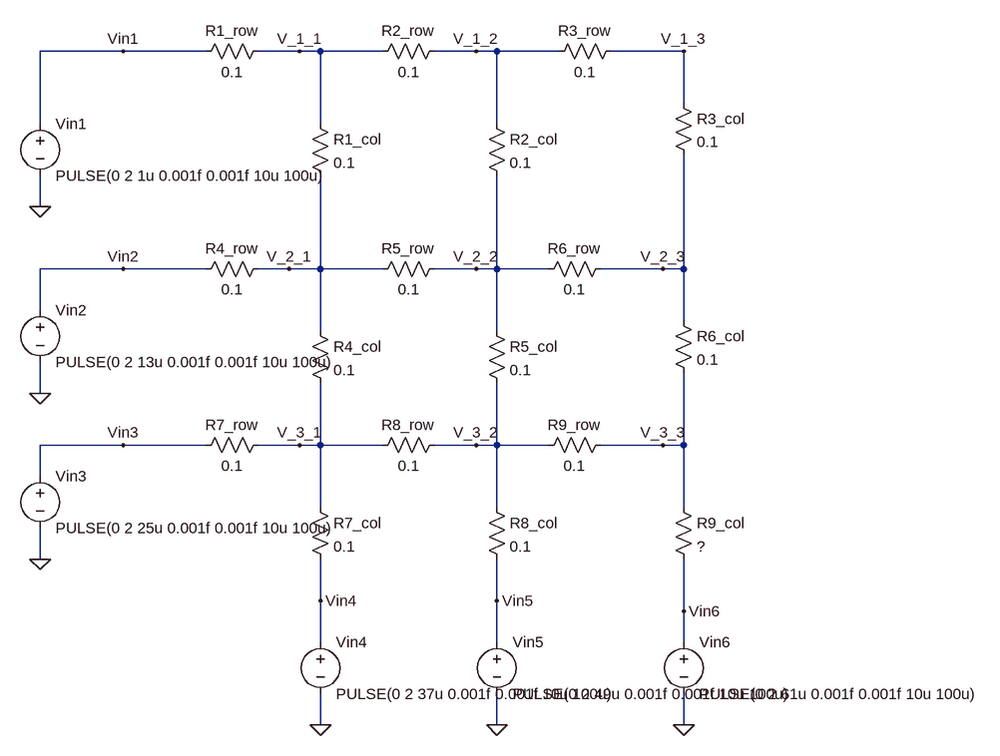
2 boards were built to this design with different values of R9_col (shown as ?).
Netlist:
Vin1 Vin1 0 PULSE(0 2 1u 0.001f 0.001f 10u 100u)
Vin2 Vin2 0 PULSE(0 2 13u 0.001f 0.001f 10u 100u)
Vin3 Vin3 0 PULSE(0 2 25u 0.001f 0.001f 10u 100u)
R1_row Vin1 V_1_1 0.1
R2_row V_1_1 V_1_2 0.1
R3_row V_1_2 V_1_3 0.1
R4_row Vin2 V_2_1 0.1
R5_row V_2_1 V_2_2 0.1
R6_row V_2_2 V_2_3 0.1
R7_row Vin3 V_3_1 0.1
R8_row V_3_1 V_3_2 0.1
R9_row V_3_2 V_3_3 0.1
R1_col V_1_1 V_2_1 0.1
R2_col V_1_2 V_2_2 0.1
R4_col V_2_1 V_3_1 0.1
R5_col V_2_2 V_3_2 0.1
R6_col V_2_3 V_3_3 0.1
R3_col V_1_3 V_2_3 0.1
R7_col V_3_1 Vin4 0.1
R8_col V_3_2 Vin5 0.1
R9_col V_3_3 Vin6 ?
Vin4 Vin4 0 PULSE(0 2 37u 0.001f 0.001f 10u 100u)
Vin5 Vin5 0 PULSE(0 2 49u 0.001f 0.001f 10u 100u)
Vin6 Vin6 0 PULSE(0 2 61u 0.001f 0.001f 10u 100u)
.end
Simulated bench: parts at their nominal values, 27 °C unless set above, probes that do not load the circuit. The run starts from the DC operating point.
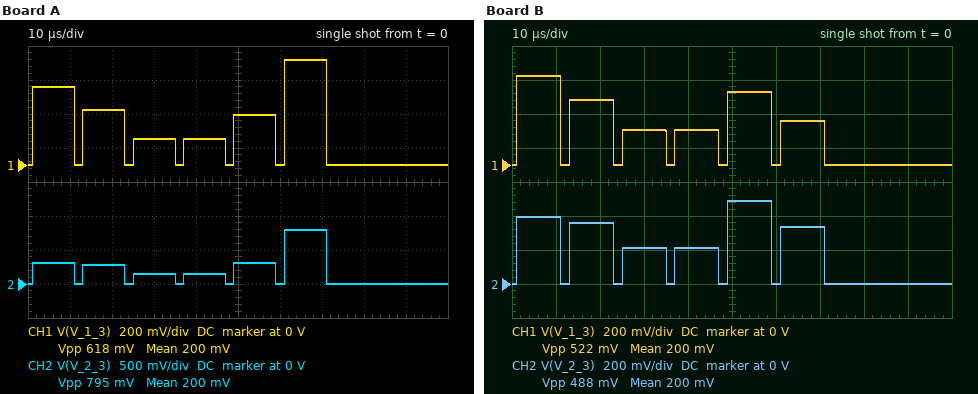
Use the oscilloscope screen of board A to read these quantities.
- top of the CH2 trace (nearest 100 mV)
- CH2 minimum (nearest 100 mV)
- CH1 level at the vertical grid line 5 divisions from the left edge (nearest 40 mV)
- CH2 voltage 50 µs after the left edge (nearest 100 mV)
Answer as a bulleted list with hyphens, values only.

- 800 mV
- 0 V
- 280 mV
- 300 mV
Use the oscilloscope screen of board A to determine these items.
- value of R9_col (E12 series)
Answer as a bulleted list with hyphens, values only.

- 0.056 Ω
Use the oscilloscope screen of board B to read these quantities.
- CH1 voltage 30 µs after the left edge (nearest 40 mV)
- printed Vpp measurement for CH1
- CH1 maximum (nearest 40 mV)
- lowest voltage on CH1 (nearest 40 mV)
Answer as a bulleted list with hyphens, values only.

- 200 mV
- 522 mV
- 520 mV
- 0 V
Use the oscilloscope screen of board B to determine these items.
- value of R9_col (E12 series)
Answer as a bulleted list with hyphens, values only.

- 0.27 Ω
